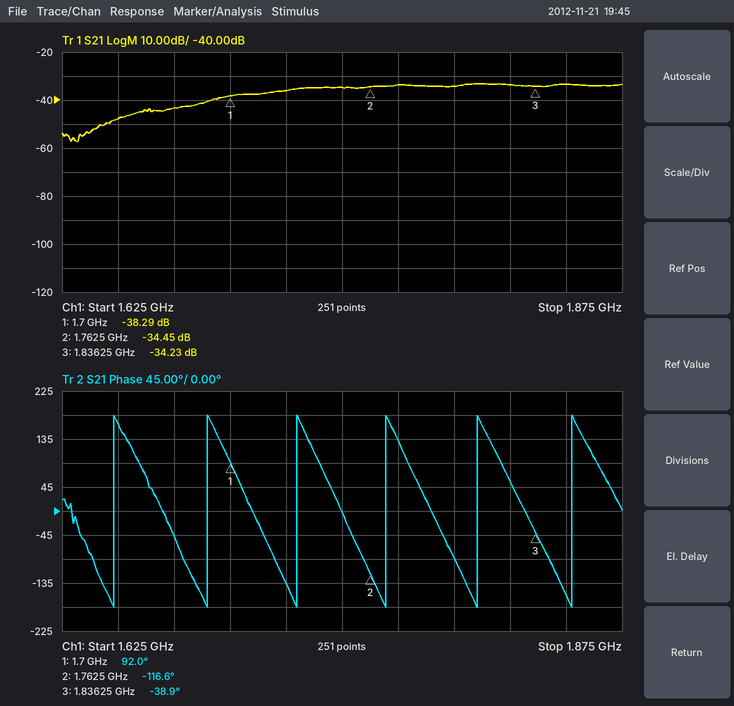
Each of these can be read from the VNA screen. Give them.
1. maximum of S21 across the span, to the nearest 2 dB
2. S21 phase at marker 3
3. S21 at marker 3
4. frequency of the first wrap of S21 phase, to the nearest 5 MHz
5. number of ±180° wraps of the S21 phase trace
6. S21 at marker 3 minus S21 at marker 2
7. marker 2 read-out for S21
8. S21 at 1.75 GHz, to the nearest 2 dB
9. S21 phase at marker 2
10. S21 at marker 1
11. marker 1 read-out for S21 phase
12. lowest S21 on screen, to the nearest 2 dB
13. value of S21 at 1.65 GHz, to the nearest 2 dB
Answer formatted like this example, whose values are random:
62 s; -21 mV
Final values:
-34 dB; -38.9°; -34.23 dB; 1.650 GHz; 6; 0.22 dB; -34.45 dB; -34 dB; -116.6°; -38.29 dB; 92.0°; -58 dB; -48 dB
